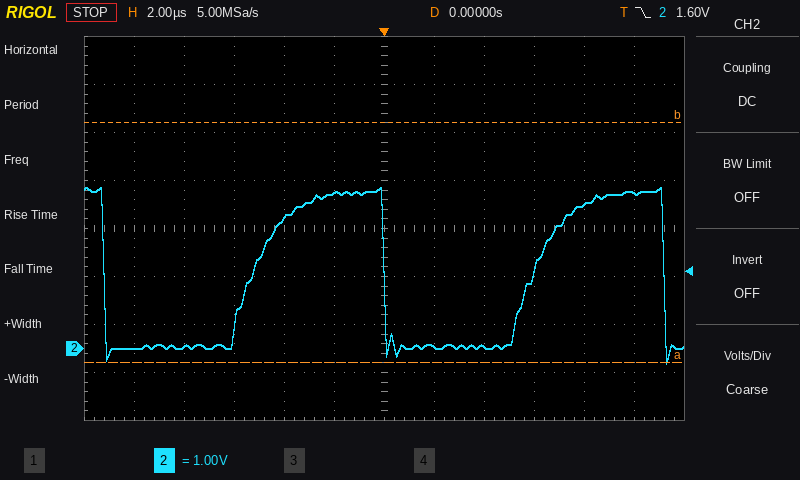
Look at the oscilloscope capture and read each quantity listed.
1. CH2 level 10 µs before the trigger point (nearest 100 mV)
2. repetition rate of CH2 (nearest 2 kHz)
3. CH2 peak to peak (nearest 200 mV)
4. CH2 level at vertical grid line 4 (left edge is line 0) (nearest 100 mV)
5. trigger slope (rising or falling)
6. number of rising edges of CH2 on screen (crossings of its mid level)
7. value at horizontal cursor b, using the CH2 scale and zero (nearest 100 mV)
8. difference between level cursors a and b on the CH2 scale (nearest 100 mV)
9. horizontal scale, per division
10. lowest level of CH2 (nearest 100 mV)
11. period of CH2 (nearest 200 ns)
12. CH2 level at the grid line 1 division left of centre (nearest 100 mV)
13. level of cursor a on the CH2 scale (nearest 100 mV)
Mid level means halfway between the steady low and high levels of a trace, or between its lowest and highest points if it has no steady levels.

0.0 V
90 kHz
3.6 V
2.7 V
falling
2
4.7 V
5.0 V
2 µs
-300 mV
11.2 µs
3.2 V
-300 mV
